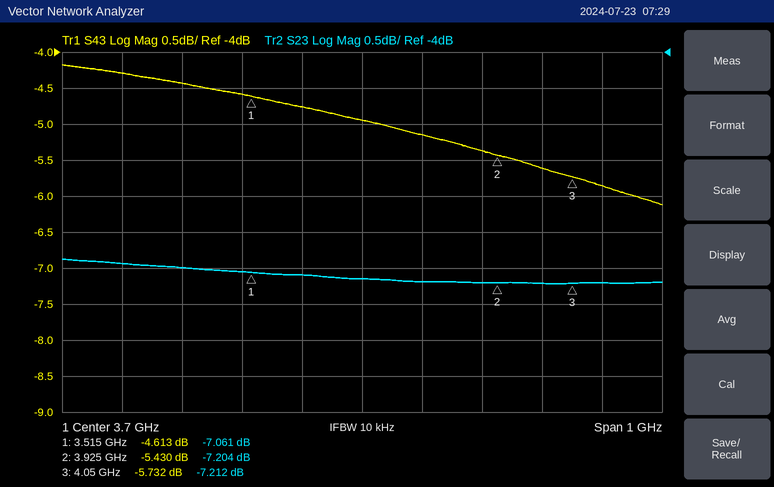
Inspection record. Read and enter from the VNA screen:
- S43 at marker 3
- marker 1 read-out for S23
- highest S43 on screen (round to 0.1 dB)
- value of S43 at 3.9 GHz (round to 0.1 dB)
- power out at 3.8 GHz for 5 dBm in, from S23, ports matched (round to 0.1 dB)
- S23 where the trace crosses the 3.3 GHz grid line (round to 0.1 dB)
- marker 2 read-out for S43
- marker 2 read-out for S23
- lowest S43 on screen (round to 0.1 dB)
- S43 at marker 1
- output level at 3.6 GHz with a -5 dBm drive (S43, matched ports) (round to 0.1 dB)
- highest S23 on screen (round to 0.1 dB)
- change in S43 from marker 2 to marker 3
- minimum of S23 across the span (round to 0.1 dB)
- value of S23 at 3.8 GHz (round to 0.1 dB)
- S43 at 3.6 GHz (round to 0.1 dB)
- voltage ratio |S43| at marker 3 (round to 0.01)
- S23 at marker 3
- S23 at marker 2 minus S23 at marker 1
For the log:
-5.732 dB
-7.061 dB
-4.2 dB
-5.4 dB
-2.2 dBm
-6.9 dB
-5.430 dB
-7.204 dB
-6.1 dB
-4.613 dB
-9.8 dBm
-6.9 dB
-0.302 dB
-7.2 dB
-7.2 dB
-4.8 dB
0.52
-7.212 dB
-0.143 dB
